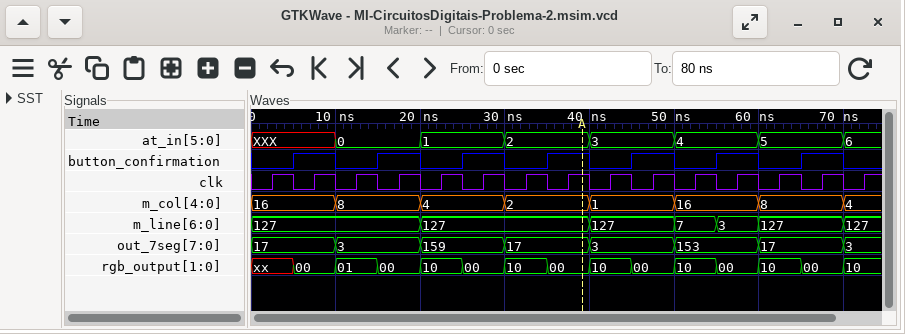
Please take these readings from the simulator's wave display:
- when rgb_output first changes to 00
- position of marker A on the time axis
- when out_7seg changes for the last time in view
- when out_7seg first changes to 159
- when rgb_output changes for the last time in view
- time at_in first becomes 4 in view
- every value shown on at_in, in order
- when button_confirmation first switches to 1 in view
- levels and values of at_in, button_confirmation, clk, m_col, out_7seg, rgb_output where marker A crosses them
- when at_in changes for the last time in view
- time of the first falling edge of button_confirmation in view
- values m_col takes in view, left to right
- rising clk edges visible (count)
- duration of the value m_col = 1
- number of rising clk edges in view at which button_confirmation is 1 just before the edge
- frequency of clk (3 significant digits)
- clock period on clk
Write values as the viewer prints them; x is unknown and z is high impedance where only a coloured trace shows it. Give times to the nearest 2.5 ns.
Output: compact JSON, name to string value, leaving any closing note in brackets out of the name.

{"when rgb_output first changes to 00": "5 ns", "position of marker A on the time axis": "40 ns", "when out_7seg changes for the last time in view": "70 ns", "when out_7seg first changes to 159": "20 ns", "when rgb_output changes for the last time in view": "70 ns", "time at_in first becomes 4 in view": "50 ns", "every value shown on at_in, in order": "XXX, 0, 1, 2, 3, 4, 5, 6", "when button_confirmation first switches to 1 in view": "5 ns", "levels and values of at_in, button_confirmation, clk, m_col, out_7seg, rgb_output where marker A crosses them": "at_in=2, button_confirmation=1, clk=1, m_col=2, out_7seg=17, rgb_output=00", "when at_in changes for the last time in view": "70 ns", "time of the first falling edge of button_confirmation in view": "10 ns", "values m_col takes in view, left to right": "16, 8, 4, 2, 1, 16, 8, 4", "rising clk edges visible": "15", "duration of the value m_col = 1": "10 ns", "number of rising clk edges in view at which button_confirmation is 1 just before the edge": "7", "frequency of clk": "200 MHz", "clock period on clk": "5 ns"}
